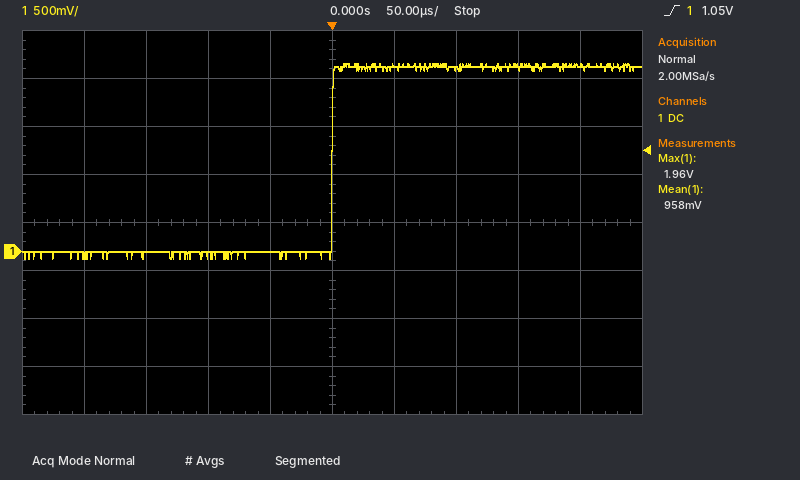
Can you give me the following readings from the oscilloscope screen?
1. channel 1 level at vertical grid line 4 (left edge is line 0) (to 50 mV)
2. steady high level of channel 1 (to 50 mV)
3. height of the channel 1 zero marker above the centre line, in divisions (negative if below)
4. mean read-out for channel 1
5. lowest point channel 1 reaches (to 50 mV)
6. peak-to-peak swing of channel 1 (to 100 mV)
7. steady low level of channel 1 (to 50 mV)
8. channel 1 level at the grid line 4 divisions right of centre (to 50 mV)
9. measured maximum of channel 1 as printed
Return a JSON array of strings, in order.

["0 mV", "1.90 V", "-0.6 div", "958 mV", "-100 mV", "2.00 V", "0 mV", "1.95 V", "1.96 V"]
